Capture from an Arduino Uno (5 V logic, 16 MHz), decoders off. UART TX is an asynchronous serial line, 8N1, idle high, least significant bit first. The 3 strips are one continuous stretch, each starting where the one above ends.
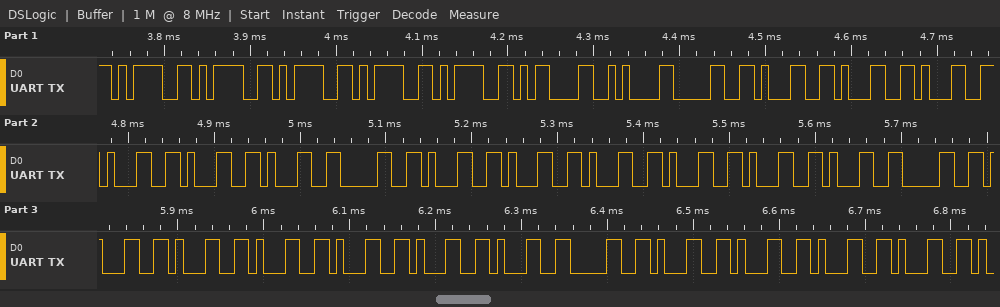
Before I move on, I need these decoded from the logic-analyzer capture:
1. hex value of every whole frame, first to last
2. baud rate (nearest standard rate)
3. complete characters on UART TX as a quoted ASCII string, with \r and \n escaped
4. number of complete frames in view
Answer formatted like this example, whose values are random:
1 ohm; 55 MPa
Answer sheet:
0x3D 0x3D 0x3D 0x3D 0x3D 0x0D 0x0A 0x30 0x31 0x31 0x31 0x31 0x31 0x31 0x30 0x31 0x31 0x31 0x31 0x31 0x31 0x30 0x31 0x31 0x31 0x31 0x31 0x31 0x30 0x31 0x31 0x31 0x31; 115200 baud; "=====\r\n01111110111111011111101111"; 33
